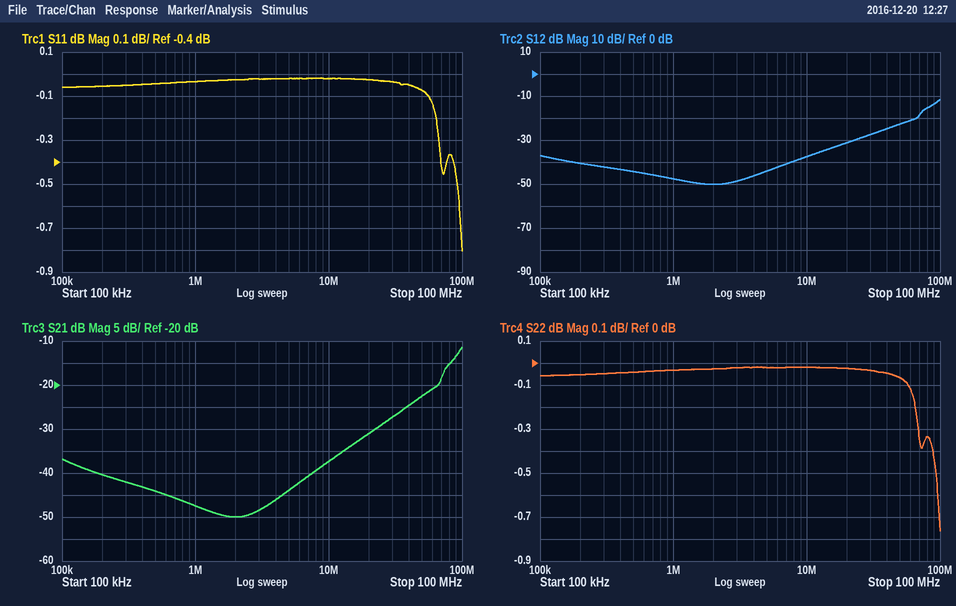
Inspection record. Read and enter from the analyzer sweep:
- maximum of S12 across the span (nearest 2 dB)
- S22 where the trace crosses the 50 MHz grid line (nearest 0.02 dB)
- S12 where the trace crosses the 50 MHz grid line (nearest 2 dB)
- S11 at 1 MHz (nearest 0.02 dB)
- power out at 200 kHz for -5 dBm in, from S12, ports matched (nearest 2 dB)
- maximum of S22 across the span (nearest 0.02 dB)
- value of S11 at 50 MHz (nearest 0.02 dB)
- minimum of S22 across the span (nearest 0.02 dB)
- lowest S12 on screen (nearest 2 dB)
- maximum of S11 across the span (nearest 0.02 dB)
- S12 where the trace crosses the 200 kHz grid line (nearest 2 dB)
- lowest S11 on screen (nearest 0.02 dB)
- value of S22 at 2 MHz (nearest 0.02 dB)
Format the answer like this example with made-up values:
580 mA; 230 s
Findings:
-12 dB; -0.06 dB; -22 dB; -0.04 dB; -46 dBm; -0.02 dB; -0.08 dB; -0.76 dB; -50 dB; -0.02 dB; -40 dB; -0.80 dB; -0.02 dB
